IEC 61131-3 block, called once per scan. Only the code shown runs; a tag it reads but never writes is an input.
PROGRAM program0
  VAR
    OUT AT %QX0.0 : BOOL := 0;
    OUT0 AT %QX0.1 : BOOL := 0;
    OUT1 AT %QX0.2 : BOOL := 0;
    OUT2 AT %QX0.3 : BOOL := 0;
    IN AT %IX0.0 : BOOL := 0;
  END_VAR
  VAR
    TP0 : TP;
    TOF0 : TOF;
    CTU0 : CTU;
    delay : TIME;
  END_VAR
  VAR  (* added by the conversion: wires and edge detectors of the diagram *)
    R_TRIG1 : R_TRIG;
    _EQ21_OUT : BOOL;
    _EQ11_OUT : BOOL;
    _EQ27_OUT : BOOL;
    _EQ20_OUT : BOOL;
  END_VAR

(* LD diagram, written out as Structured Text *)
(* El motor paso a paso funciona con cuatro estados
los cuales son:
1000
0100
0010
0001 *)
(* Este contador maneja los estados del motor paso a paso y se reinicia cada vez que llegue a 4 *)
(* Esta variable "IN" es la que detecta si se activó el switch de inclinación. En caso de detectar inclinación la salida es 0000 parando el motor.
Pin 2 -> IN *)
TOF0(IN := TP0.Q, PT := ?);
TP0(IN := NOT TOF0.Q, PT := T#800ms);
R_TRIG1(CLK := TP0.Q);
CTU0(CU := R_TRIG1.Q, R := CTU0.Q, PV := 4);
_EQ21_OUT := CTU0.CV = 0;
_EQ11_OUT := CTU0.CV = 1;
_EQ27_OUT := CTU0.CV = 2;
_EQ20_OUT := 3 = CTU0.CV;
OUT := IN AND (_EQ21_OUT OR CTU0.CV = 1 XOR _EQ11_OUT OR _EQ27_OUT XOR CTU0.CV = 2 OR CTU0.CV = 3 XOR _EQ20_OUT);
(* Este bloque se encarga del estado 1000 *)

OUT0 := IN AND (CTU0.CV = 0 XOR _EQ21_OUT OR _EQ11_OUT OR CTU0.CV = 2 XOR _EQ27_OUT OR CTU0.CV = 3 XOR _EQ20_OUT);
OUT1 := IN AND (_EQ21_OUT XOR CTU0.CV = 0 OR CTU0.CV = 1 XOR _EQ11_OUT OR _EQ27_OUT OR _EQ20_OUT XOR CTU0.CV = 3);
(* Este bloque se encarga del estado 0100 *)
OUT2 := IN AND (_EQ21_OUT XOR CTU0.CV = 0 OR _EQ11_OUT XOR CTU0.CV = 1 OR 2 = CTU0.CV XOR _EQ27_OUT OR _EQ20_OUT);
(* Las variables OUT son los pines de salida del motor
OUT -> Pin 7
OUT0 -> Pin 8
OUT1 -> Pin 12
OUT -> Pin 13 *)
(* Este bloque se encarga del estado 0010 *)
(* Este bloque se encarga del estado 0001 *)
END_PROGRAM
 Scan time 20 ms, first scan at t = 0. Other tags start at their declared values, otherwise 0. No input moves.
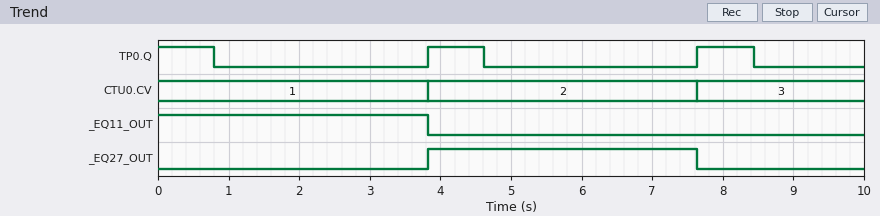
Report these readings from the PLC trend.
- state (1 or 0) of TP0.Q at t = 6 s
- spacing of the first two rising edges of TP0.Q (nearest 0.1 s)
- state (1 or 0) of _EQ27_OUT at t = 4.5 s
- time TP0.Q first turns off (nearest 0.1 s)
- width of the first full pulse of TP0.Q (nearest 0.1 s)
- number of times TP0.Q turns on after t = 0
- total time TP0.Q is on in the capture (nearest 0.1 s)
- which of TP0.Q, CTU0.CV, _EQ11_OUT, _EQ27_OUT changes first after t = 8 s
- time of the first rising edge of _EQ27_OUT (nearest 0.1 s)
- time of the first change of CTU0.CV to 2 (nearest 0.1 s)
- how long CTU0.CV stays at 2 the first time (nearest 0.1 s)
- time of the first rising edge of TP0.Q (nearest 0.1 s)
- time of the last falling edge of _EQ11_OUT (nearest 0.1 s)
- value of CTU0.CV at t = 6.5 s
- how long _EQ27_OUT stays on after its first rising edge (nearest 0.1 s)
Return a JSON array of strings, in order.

["0", "3.8 s", "1", "0.8 s", "0.8 s", "2", "2.4 s", "TP0.Q", "3.8 s", "3.8 s", "3.8 s", "3.8 s", "3.8 s", "2", "3.8 s"]
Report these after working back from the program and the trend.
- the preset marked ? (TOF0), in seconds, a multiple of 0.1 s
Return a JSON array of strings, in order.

["3.0 s"]
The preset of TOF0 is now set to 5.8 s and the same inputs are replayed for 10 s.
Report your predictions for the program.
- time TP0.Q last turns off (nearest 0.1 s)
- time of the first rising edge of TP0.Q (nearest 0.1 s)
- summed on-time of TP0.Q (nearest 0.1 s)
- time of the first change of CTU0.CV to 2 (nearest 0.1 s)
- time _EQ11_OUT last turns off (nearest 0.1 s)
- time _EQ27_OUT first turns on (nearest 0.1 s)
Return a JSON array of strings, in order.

["7.4 s", "6.6 s", "1.6 s", "6.6 s", "6.6 s", "6.6 s"]
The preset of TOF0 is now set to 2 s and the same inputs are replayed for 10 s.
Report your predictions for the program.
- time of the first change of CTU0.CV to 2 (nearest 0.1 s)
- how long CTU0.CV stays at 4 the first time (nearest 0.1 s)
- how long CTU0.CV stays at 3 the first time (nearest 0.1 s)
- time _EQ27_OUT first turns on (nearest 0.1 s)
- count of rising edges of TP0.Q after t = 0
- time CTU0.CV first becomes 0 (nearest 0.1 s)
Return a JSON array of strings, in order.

["2.8 s", "0.0 s", "2.8 s", "2.8 s", "3", "8.5 s"]
